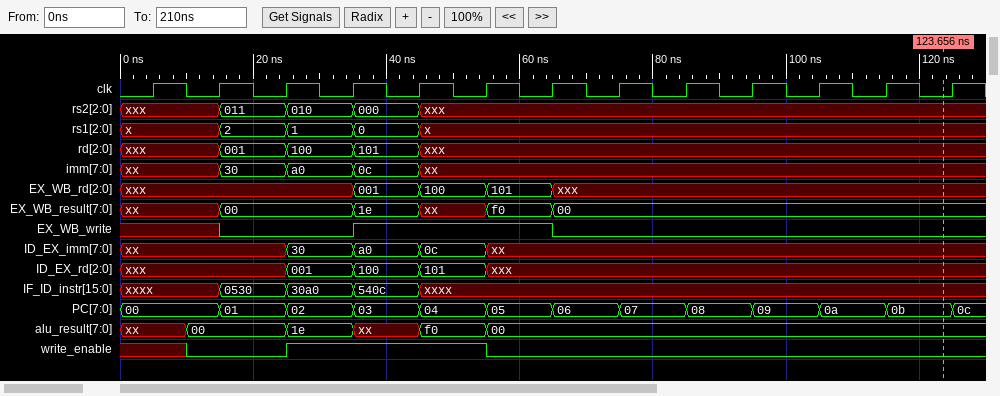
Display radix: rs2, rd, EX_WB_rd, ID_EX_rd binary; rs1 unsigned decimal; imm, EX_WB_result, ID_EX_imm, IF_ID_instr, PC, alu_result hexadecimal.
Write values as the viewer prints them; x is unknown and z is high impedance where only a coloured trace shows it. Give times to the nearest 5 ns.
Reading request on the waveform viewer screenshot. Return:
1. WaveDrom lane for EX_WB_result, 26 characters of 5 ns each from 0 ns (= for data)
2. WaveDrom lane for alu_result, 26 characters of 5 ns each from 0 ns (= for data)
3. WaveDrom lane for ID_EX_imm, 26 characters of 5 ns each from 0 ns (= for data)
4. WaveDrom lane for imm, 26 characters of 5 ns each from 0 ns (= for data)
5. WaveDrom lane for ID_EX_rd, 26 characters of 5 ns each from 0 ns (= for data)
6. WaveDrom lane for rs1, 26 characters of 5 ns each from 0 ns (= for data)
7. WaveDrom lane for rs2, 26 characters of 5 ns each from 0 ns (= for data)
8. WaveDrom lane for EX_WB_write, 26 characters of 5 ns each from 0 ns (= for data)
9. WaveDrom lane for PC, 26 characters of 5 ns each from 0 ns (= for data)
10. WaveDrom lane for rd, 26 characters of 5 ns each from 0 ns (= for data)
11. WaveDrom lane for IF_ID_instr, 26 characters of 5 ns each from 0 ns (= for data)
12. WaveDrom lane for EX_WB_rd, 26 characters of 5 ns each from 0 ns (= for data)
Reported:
{name: 'EX_WB_result', wave: 'x..=...=.x.=.=............', data: '00 1e f0 00'}
{name: 'alu_result', wave: 'x.=..=.x.=.=..............', data: '00 1e f0 00'}
{name: 'ID_EX_imm', wave: 'x....=.=.=.x..............', data: '30 a0 0c'}
{name: 'imm', wave: 'x..=.=.=.x................', data: '30 a0 0c'}
{name: 'ID_EX_rd', wave: 'x....=.=.=.x..............', data: '001 100 101'}
{name: 'rs1', wave: 'x..=.=.=.x................', data: '2 1 0'}
{name: 'rs2', wave: 'x..=.=.=.x................', data: '011 010 000'}
{name: 'EX_WB_write', wave: 'x..0...1.....0............'}
{name: 'PC', wave: '=..=.=.=.=.=.=.=.=.=.=.=.=', data: '00 01 02 03 04 05 06 07 08 09 0a 0b 0c'}
{name: 'rd', wave: 'x..=.=.=.x................', data: '001 100 101'}
{name: 'IF_ID_instr', wave: 'x..=.=.=.x................', data: '0530 30a0 540c'}
{name: 'EX_WB_rd', wave: 'x......=.=.=.x............', data: '001 100 101'}
